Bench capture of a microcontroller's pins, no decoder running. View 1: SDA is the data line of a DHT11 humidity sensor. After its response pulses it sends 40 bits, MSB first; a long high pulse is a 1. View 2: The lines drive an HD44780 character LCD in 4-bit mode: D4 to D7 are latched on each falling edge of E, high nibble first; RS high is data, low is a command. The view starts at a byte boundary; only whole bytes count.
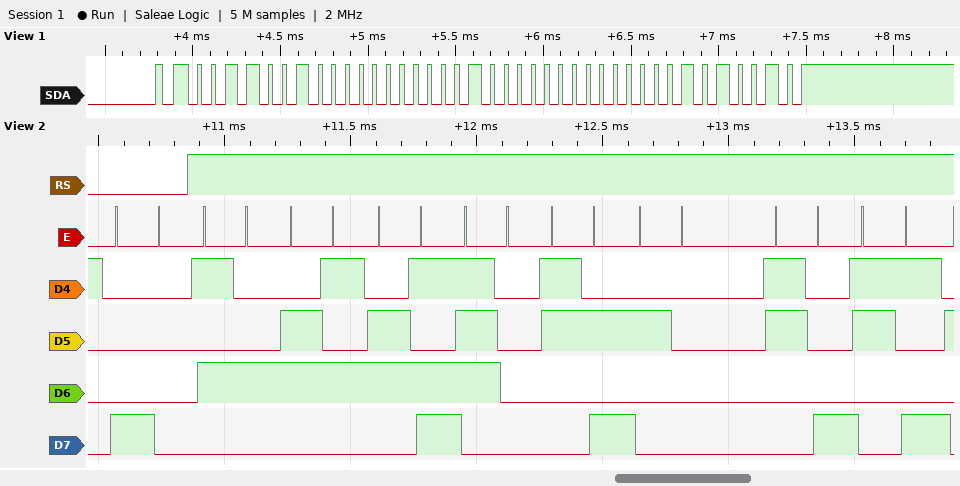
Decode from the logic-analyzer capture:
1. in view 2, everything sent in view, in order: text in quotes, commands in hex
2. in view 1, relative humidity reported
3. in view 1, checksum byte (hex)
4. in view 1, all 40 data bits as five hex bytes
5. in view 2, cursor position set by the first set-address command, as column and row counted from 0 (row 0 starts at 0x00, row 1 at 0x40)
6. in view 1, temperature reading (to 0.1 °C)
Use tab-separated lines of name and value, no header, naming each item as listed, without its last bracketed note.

in view 2, everything sent in view, in order: text in quotes, commands in hex	0x80 "Temp: 89"
in view 1, relative humidity reported	50 %
in view 1, checksum byte	0x52
in view 1, all 40 data bits as five hex bytes	32 00 20 00 52
in view 2, cursor position set by the first set-address command, as column and row counted from 0	column 0, row 0
in view 1, temperature reading	32.0 °C
